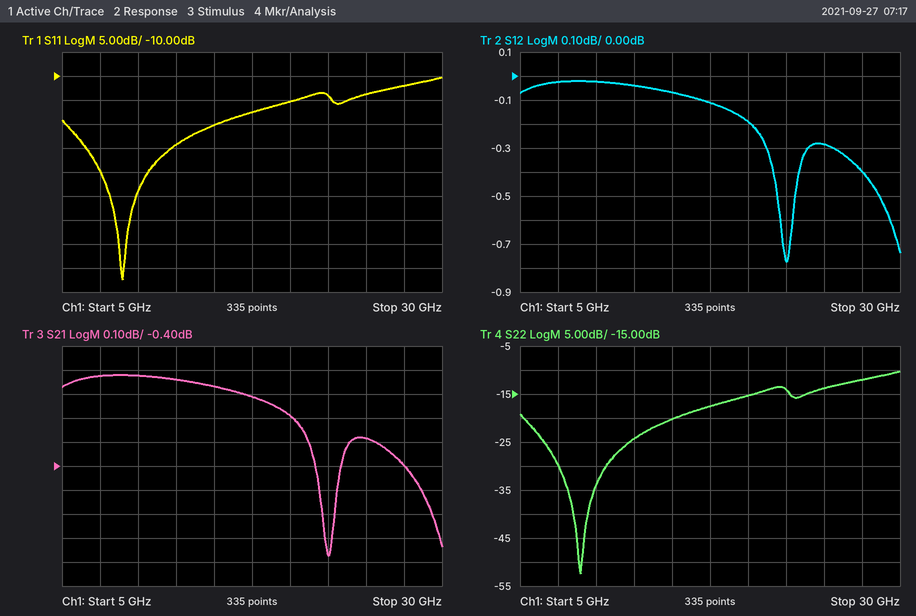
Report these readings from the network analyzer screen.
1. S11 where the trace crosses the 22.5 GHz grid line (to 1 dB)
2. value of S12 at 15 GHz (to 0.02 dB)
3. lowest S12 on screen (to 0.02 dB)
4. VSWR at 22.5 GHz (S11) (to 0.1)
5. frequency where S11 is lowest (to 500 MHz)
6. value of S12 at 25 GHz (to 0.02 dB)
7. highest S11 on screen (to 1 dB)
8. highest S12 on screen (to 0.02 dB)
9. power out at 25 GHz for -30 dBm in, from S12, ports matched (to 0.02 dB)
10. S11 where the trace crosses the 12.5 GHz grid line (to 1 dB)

-14 dB
-0.06 dB
-0.78 dB
1.5
9.0 GHz
-0.28 dB
-10 dB
-0.02 dB
-30.28 dBm
-24 dB
